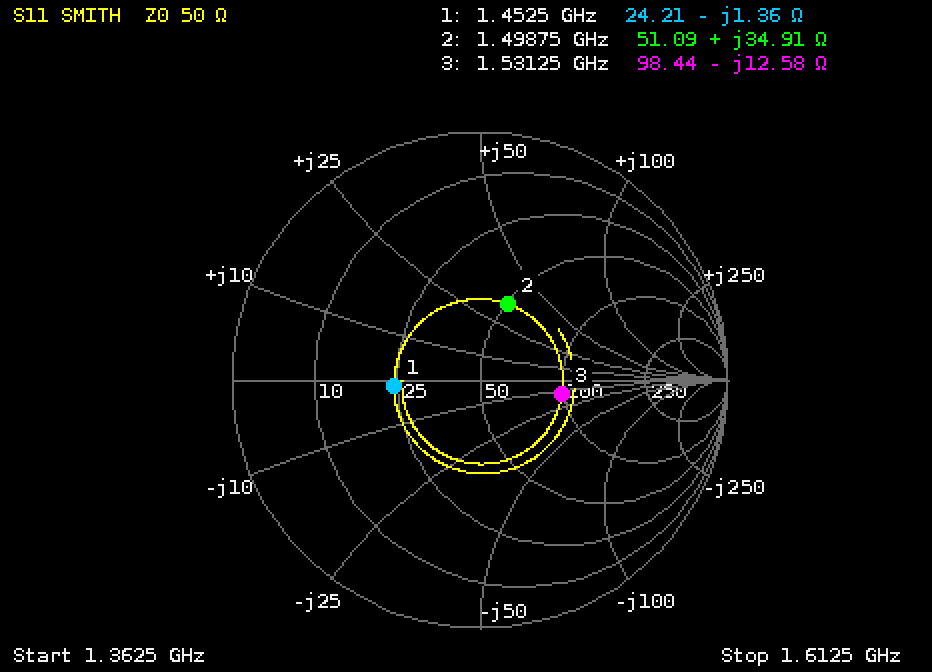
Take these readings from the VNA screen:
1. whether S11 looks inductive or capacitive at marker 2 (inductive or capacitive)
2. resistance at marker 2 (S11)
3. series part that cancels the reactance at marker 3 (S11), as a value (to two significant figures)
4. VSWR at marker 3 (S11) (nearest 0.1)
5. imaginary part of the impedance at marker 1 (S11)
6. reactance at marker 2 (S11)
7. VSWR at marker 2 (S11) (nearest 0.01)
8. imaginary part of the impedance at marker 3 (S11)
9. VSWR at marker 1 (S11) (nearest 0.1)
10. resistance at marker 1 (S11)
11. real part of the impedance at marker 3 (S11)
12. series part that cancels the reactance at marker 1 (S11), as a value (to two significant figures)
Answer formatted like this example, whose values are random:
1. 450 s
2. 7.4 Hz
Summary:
1. inductive
2. 51.09 Ω
3. 1.3 nH
4. 2.0
5. -1.36 Ω
6. +34.91 Ω
7. 1.97
8. -12.58 Ω
9. 2.1
10. 24.21 Ω
11. 98.44 Ω
12. 150 pH
